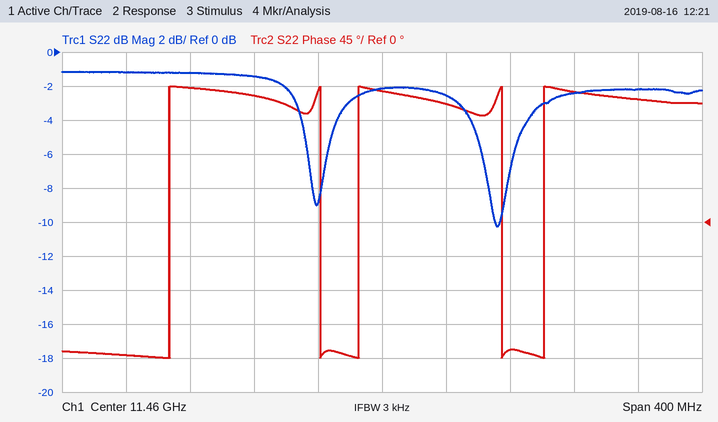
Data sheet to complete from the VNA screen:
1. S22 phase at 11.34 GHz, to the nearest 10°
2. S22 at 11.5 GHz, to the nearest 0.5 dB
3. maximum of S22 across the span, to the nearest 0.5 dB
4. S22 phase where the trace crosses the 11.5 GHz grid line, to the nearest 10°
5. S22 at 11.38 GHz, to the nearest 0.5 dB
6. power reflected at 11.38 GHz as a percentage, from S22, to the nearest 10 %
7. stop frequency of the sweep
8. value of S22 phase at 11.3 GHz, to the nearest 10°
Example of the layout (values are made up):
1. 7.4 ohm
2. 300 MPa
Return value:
1. 180°
2. -2.5 dB
3. -1.0 dB
4. 160°
5. -1.5 dB
6. 70 %
7. 11.66 GHz
8. -180°
